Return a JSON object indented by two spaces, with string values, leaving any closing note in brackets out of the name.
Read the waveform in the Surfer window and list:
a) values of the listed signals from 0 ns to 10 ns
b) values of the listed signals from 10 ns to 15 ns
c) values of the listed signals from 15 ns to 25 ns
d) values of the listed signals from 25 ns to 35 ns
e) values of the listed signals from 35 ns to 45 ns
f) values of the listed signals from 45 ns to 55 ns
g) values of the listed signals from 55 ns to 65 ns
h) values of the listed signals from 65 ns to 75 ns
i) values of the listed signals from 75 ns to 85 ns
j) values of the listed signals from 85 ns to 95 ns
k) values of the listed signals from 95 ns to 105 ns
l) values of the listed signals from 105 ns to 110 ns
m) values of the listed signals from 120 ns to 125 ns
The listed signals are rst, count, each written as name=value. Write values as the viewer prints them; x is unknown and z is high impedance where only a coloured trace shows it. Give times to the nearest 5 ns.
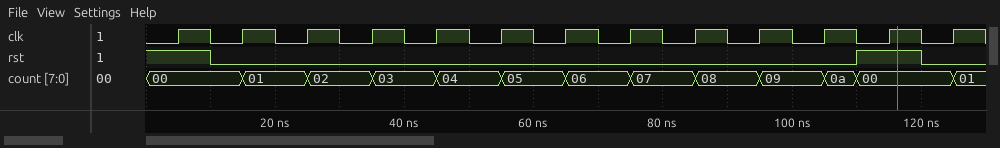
{
  "values of the listed signals from 0 ns to 10 ns": "rst=1, count=00",
  "values of the listed signals from 10 ns to 15 ns": "rst=0, count=00",
  "values of the listed signals from 15 ns to 25 ns": "rst=0, count=01",
  "values of the listed signals from 25 ns to 35 ns": "rst=0, count=02",
  "values of the listed signals from 35 ns to 45 ns": "rst=0, count=03",
  "values of the listed signals from 45 ns to 55 ns": "rst=0, count=04",
  "values of the listed signals from 55 ns to 65 ns": "rst=0, count=05",
  "values of the listed signals from 65 ns to 75 ns": "rst=0, count=06",
  "values of the listed signals from 75 ns to 85 ns": "rst=0, count=07",
  "values of the listed signals from 85 ns to 95 ns": "rst=0, count=08",
  "values of the listed signals from 95 ns to 105 ns": "rst=0, count=09",
  "values of the listed signals from 105 ns to 110 ns": "rst=0, count=0a",
  "values of the listed signals from 120 ns to 125 ns": "rst=0, count=00"
}
